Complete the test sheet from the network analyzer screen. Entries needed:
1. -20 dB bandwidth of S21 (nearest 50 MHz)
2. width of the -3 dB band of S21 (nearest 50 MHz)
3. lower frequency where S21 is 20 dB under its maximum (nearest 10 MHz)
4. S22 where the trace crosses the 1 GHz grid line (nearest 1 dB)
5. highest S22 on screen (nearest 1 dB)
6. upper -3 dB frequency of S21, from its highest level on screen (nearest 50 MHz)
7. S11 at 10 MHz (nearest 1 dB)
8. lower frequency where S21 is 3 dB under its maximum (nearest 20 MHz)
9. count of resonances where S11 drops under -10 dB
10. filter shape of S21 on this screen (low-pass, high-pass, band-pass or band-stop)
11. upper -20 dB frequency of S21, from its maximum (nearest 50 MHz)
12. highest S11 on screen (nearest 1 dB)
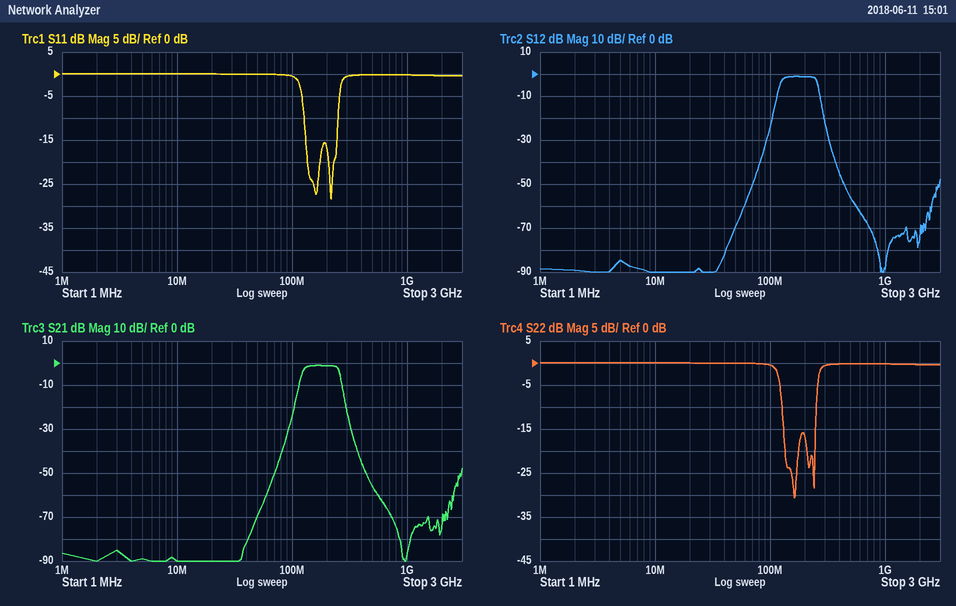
200 MHz
150 MHz
100 MHz
0 dB
0 dB
250 MHz
0 dB
120 MHz
2
band-pass
300 MHz
0 dB
